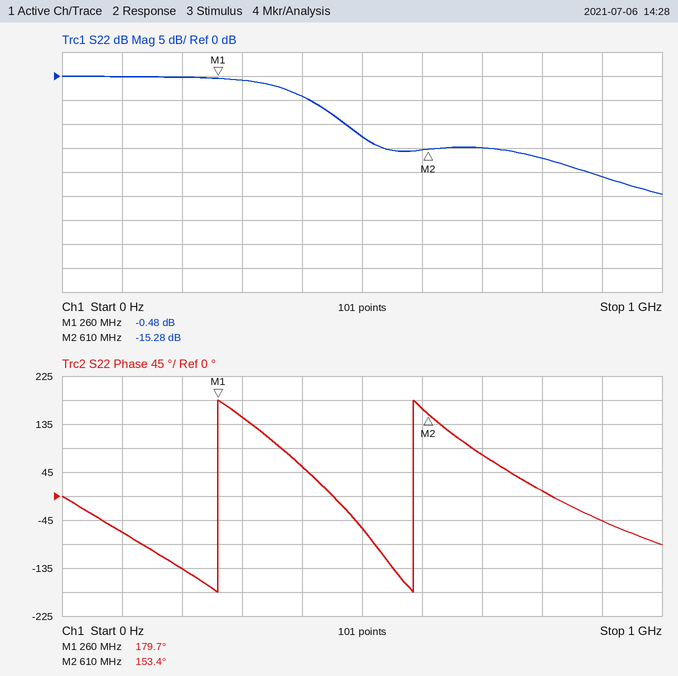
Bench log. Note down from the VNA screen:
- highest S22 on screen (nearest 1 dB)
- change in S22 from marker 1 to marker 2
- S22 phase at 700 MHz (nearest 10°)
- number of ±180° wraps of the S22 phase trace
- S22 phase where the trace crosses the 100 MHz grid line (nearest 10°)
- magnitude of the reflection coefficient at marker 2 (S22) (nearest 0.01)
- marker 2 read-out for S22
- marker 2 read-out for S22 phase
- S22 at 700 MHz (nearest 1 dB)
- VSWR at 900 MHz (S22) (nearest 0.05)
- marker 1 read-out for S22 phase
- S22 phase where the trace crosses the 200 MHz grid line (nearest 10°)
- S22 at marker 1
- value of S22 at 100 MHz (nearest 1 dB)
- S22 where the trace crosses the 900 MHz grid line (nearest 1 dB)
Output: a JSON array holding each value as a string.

["0 dB", "-14.80 dB", "80°", "2", "-70°", "0.17", "-15.28 dB", "153.4°", "-15 dB", "1.20", "179.7°", "-140°", "-0.48 dB", "0 dB", "-21 dB"]
